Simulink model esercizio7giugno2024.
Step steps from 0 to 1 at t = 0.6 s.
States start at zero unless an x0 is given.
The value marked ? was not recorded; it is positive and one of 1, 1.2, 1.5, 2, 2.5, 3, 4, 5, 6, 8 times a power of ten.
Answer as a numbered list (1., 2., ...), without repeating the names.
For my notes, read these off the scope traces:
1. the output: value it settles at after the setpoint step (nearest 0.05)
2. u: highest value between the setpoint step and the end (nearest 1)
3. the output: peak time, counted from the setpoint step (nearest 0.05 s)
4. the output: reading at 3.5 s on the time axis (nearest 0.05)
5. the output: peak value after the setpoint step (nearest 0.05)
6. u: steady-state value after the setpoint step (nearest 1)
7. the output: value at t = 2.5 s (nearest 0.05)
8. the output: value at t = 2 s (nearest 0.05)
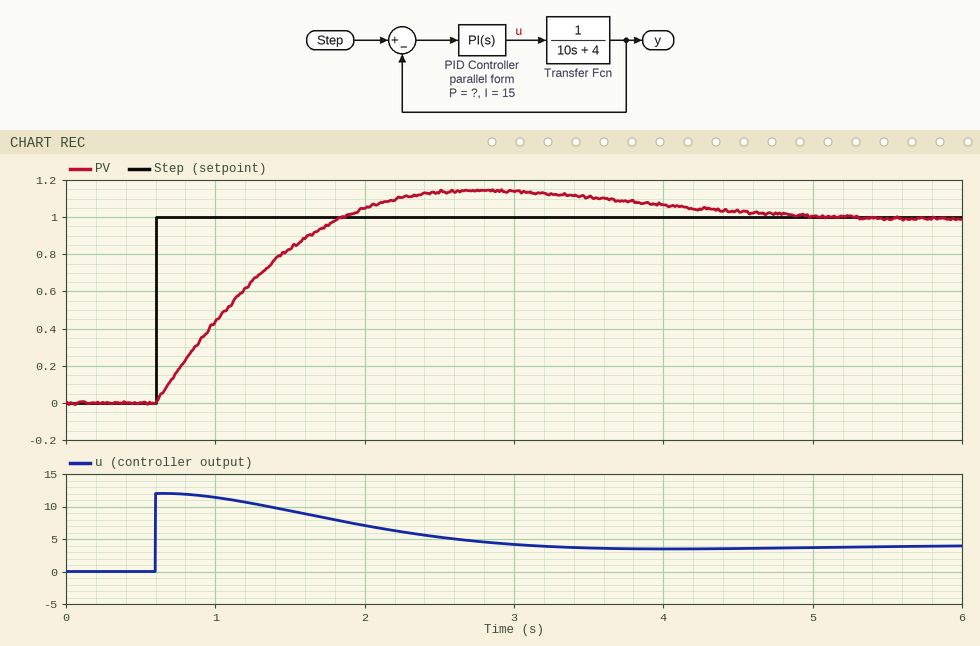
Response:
1. 1.00
2. 12
3. 2.20 s
4. 1.10
5. 1.15
6. 4
7. 1.15
8. 1.05
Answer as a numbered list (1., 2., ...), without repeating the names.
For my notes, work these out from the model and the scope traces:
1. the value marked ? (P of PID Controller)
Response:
1. 12
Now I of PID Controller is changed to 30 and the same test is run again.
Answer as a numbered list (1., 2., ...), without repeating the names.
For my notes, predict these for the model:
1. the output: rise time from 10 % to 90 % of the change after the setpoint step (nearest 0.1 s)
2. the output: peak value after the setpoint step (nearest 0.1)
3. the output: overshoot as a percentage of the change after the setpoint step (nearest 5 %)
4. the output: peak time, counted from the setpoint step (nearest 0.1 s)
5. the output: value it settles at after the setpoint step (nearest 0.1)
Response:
1. 0.7 s
2. 1.3
3. 25 %
4. 1.6 s
5. 1.0
